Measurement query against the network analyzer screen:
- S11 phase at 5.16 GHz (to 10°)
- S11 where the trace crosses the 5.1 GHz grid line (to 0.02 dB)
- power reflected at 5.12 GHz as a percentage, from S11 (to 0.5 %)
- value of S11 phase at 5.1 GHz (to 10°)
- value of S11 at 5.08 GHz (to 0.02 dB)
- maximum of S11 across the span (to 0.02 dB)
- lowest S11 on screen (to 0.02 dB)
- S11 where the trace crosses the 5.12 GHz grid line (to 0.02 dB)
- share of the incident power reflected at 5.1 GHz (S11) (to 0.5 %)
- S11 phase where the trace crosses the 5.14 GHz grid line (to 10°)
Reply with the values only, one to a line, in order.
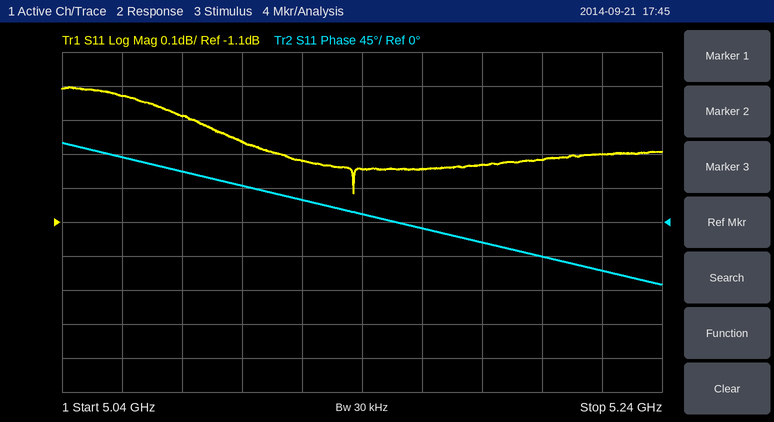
-10°
-0.86 dB
81.0 %
50°
-0.78 dB
-0.70 dB
-1.02 dB
-0.92 dB
82.0 %
10°
